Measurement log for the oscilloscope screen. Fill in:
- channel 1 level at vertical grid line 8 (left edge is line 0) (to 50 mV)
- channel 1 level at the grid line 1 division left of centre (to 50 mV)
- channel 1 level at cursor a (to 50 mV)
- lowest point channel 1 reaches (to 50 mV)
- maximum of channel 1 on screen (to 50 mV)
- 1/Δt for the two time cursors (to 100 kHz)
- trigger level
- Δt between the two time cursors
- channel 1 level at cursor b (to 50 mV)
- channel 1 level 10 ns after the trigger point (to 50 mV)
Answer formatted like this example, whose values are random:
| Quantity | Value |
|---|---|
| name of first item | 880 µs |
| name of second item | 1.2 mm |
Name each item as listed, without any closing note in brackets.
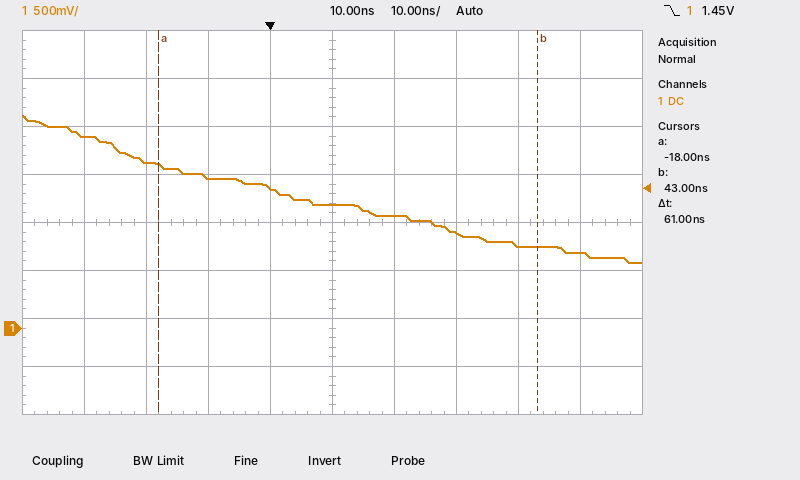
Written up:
| Quantity | Value |
|---|---|
| channel 1 level at vertical grid line 8 (left edge is line 0) | 850 mV |
| channel 1 level at the grid line 1 division left of centre | 1.45 V |
| channel 1 level at cursor a | 1.70 V |
| lowest point channel 1 reaches | 700 mV |
| maximum of channel 1 on screen | 2.20 V |
| 1/Δt for the two time cursors | 16.4 MHz |
| trigger level | 1.45 V |
| Δt between the two time cursors | 61 ns |
| channel 1 level at cursor b | 850 mV |
| channel 1 level 10 ns after the trigger point | 1.30 V |
